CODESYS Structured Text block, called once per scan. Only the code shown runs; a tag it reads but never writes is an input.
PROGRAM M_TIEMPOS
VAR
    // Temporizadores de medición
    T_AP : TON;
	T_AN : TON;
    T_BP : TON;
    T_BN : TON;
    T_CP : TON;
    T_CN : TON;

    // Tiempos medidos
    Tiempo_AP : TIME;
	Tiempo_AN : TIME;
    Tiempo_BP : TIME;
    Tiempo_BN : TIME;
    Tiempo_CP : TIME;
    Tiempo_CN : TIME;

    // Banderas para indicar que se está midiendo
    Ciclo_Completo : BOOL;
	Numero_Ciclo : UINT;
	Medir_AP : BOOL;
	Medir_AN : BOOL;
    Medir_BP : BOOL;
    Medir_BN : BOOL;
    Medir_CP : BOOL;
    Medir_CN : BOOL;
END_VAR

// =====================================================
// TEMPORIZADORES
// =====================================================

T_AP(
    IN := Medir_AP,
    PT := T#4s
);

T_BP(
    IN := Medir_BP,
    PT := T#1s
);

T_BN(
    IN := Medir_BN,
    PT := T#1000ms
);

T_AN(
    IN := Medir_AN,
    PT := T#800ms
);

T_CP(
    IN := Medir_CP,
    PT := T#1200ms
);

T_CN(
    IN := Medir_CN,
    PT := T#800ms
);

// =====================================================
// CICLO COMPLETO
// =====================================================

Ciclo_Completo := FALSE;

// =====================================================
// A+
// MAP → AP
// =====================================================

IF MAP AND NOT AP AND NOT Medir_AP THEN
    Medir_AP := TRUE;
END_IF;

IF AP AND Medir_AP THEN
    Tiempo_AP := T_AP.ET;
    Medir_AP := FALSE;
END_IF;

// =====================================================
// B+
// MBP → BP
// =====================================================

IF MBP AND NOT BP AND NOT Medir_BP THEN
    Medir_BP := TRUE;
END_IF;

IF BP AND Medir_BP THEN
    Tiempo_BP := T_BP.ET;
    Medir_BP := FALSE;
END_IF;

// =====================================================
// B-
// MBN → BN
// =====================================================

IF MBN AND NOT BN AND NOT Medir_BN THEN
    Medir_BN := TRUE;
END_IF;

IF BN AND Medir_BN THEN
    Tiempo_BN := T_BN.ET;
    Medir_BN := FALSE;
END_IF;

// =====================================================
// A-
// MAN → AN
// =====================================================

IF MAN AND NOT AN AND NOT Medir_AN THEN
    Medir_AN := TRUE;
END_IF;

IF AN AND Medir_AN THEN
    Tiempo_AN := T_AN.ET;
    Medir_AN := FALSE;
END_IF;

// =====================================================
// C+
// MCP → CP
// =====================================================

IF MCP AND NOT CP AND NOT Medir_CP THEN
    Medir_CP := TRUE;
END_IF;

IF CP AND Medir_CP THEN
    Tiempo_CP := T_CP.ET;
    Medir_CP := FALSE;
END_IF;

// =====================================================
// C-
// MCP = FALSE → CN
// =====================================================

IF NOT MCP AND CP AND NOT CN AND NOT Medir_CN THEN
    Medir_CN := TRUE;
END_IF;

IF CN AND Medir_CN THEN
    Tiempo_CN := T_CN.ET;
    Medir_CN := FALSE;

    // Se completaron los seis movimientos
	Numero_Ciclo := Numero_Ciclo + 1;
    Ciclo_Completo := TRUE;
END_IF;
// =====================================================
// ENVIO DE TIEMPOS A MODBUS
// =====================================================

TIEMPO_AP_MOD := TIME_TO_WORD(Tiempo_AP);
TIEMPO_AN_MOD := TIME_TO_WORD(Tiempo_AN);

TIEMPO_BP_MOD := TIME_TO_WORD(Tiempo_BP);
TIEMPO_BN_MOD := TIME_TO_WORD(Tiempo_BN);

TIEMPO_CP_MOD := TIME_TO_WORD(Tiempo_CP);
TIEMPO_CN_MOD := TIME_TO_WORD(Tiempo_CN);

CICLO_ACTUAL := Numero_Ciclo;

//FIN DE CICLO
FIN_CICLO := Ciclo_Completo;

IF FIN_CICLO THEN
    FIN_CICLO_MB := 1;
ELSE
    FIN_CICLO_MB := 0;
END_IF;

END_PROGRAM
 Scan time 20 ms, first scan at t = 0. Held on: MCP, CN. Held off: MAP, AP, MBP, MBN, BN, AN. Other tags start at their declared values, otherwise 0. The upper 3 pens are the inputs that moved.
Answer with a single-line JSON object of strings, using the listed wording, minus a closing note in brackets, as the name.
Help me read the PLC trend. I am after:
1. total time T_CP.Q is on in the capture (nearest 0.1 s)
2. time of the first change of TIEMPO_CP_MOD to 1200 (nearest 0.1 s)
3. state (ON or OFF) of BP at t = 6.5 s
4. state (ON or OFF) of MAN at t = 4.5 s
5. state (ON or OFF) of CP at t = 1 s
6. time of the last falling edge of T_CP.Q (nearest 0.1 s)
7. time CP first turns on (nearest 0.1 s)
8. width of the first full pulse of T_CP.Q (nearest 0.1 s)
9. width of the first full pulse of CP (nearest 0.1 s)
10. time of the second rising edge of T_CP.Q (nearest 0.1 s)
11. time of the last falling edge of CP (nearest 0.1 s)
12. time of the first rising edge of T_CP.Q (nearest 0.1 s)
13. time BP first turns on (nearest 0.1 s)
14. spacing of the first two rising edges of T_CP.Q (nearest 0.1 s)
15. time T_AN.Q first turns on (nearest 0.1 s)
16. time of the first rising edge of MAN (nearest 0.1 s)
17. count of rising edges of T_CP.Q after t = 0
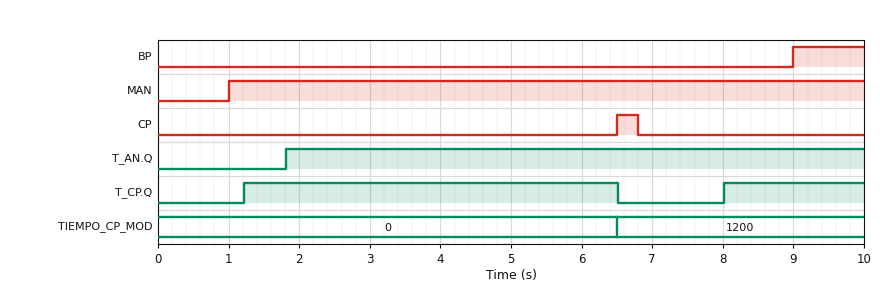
{"total time T_CP.Q is on in the capture": "7.3 s", "time of the first change of TIEMPO_CP_MOD to 1200": "6.5 s", "state (ON or OFF) of BP at t = 6.5 s": "OFF", "state (ON or OFF) of MAN at t = 4.5 s": "ON", "state (ON or OFF) of CP at t = 1 s": "OFF", "time of the last falling edge of T_CP.Q": "6.5 s", "time CP first turns on": "6.5 s", "width of the first full pulse of T_CP.Q": "5.3 s", "width of the first full pulse of CP": "0.3 s", "time of the second rising edge of T_CP.Q": "8.0 s", "time of the last falling edge of CP": "6.8 s", "time of the first rising edge of T_CP.Q": "1.2 s", "time BP first turns on": "9.0 s", "spacing of the first two rising edges of T_CP.Q": "6.8 s", "time T_AN.Q first turns on": "1.8 s", "time of the first rising edge of MAN": "1.0 s", "count of rising edges of T_CP.Q after t = 0": "2"}
